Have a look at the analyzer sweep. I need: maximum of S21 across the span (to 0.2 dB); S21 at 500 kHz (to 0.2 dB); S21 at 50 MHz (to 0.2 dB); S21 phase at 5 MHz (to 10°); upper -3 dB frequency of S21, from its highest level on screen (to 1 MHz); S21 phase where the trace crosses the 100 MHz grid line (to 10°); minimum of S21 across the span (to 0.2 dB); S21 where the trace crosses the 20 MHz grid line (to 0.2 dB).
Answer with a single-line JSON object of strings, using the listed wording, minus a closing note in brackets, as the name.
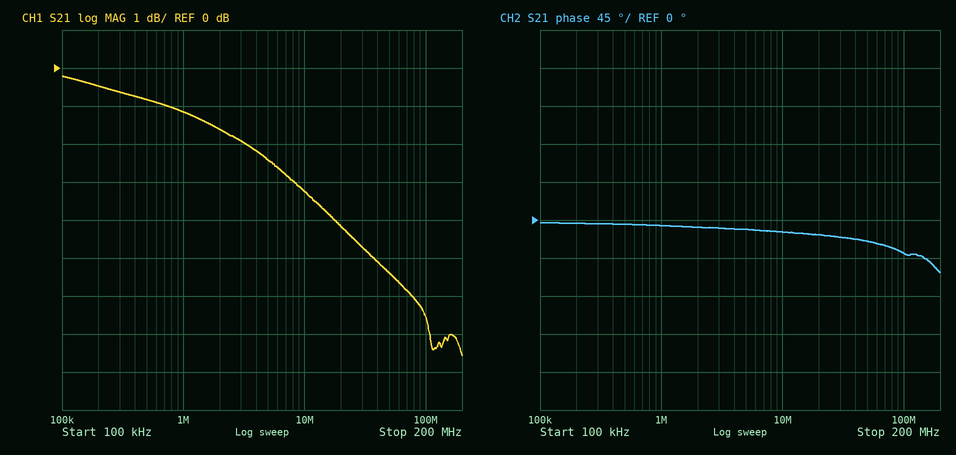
{"maximum of S21 across the span": "-0.2 dB", "S21 at 500 kHz": "-0.8 dB", "S21 at 50 MHz": "-5.4 dB", "S21 phase at 5 MHz": "-10°", "upper -3 dB frequency of S21, from its highest level on screen": "10 MHz", "S21 phase where the trace crosses the 100 MHz grid line": "-40°", "minimum of S21 across the span": "-7.6 dB", "S21 where the trace crosses the 20 MHz grid line": "-4.2 dB"}
